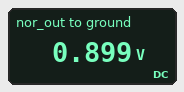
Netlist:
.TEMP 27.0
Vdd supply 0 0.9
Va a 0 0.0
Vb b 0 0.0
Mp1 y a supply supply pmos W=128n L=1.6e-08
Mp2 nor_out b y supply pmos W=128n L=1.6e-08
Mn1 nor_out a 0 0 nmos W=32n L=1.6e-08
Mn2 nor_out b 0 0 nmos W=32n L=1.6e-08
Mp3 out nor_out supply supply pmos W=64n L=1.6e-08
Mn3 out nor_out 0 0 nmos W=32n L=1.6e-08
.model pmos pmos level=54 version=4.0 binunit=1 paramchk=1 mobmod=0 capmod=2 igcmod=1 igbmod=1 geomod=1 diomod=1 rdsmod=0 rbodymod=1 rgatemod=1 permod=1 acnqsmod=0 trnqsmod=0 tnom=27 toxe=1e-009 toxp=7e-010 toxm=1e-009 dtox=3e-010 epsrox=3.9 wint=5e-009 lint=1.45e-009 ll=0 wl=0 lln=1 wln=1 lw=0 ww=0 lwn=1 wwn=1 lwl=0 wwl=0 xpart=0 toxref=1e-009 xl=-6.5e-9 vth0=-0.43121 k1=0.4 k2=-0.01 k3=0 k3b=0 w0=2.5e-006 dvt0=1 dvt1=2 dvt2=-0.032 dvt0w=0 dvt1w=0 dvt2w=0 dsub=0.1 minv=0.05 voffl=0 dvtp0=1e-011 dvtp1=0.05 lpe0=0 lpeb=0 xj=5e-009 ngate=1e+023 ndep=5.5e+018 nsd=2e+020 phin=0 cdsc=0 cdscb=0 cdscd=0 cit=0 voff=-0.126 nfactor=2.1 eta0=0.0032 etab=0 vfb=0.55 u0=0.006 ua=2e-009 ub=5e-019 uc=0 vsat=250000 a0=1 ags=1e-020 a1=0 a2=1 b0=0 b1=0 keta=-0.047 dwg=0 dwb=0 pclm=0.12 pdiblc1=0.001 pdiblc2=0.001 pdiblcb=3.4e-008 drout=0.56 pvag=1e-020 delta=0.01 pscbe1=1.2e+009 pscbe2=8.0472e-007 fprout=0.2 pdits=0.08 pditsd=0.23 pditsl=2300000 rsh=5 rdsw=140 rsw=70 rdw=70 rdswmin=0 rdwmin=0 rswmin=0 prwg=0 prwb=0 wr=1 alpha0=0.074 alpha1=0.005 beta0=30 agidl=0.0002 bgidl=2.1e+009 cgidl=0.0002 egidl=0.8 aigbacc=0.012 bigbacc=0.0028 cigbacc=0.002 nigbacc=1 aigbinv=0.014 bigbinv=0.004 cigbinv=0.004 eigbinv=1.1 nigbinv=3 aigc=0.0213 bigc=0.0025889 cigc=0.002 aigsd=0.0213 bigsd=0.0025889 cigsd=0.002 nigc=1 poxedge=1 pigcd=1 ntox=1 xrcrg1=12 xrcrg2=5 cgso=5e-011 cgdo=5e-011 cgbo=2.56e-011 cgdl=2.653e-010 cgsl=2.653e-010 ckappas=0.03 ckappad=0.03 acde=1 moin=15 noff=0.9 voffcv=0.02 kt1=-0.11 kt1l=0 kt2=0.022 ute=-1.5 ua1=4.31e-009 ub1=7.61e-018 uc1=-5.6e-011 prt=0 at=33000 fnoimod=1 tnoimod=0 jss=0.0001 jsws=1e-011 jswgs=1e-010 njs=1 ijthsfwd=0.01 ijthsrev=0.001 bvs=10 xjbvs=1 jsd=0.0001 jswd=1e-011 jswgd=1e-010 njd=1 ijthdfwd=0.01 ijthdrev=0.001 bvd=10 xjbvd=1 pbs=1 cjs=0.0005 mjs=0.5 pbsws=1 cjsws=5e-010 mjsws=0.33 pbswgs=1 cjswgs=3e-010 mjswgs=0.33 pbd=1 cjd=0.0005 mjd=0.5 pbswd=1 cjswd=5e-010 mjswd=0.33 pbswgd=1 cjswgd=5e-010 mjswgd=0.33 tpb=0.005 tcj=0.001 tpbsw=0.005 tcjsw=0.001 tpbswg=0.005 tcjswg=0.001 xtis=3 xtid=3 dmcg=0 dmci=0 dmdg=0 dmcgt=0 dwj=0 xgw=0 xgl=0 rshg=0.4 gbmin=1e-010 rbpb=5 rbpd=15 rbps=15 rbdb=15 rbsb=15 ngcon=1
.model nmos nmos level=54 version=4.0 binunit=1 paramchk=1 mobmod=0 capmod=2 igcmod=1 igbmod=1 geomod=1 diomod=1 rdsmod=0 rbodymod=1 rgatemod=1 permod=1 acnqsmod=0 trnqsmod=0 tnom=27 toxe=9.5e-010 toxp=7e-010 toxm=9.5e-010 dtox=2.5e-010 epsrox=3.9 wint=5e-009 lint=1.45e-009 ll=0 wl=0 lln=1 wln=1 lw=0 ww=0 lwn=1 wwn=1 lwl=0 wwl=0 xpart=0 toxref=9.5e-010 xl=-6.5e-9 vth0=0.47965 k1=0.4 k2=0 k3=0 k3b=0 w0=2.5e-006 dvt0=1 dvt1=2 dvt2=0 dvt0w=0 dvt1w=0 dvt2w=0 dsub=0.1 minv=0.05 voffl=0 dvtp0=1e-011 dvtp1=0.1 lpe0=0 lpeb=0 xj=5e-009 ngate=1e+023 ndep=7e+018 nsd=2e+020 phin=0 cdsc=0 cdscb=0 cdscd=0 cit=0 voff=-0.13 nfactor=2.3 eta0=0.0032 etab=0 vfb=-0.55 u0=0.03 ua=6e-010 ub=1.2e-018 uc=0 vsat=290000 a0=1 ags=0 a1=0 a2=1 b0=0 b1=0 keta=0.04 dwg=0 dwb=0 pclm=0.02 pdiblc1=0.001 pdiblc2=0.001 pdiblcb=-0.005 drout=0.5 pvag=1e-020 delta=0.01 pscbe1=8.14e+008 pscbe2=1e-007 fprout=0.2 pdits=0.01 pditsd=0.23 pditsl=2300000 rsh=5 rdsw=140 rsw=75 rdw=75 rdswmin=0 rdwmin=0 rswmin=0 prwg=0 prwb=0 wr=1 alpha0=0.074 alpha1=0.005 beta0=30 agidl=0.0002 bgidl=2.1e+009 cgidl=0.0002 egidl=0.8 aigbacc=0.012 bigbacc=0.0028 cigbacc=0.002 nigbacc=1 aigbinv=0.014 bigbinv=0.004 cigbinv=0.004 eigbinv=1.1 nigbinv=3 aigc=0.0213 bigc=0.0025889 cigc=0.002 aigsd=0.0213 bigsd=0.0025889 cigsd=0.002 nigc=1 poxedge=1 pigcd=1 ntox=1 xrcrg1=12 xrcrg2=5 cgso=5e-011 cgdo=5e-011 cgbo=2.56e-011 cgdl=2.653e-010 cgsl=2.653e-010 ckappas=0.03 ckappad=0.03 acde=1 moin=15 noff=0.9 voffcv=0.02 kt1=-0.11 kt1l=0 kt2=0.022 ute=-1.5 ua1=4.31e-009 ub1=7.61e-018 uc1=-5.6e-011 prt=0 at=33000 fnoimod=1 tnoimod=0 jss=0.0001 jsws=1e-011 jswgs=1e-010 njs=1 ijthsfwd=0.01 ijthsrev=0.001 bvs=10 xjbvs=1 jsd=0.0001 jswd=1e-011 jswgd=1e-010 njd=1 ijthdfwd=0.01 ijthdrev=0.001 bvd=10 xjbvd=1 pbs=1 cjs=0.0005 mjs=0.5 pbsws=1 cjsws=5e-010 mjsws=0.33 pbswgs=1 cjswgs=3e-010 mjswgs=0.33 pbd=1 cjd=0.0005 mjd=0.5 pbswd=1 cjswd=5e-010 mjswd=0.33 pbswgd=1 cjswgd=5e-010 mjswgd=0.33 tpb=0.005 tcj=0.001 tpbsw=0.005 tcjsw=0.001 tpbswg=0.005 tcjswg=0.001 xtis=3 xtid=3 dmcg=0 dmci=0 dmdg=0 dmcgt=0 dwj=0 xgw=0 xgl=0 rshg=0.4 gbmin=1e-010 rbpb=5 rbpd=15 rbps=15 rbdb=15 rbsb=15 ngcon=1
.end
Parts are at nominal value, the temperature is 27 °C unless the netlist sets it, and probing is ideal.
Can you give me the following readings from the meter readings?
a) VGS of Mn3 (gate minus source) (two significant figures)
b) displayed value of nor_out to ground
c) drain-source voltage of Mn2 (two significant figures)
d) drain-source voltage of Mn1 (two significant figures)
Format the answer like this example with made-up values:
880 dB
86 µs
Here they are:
900 mV
0.899 V
900 mV
900 mV
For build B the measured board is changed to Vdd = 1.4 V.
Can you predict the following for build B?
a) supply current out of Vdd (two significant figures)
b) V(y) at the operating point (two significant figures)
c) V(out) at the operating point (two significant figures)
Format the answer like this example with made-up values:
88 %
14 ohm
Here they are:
25 µA
1.4 V
120 mV
